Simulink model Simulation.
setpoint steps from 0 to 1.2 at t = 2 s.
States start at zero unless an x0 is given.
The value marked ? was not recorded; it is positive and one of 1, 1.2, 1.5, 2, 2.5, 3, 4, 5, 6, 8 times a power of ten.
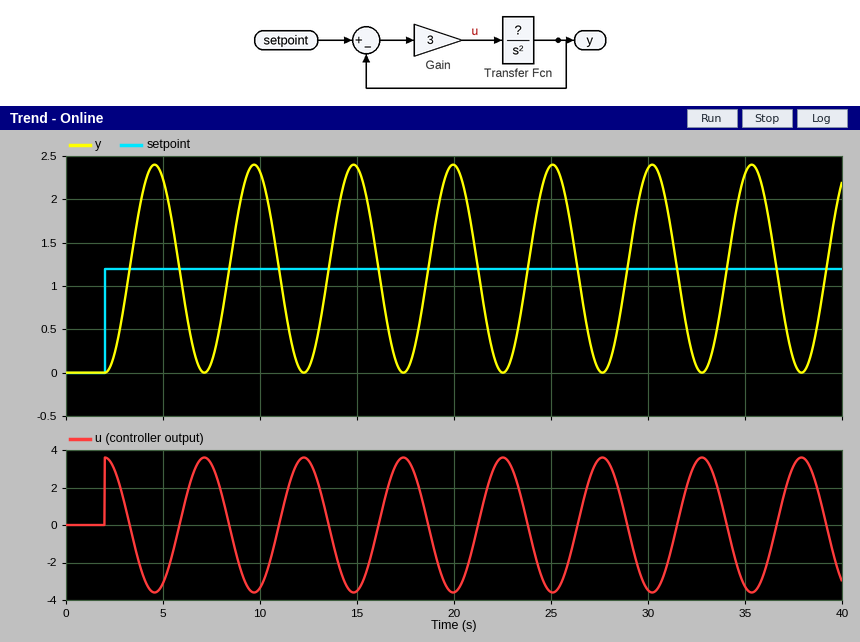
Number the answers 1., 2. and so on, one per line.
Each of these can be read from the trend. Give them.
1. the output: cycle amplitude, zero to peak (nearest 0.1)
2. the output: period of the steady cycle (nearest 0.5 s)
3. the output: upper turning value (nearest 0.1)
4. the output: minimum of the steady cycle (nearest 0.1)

1. 1.2
2. 5.0 s
3. 2.4
4. 0.0
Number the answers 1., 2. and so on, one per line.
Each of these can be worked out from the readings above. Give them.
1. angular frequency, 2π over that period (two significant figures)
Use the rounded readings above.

1. 1.3 rad/s
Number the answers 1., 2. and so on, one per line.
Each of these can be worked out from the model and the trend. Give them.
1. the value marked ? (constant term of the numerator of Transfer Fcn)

1. 0.5
